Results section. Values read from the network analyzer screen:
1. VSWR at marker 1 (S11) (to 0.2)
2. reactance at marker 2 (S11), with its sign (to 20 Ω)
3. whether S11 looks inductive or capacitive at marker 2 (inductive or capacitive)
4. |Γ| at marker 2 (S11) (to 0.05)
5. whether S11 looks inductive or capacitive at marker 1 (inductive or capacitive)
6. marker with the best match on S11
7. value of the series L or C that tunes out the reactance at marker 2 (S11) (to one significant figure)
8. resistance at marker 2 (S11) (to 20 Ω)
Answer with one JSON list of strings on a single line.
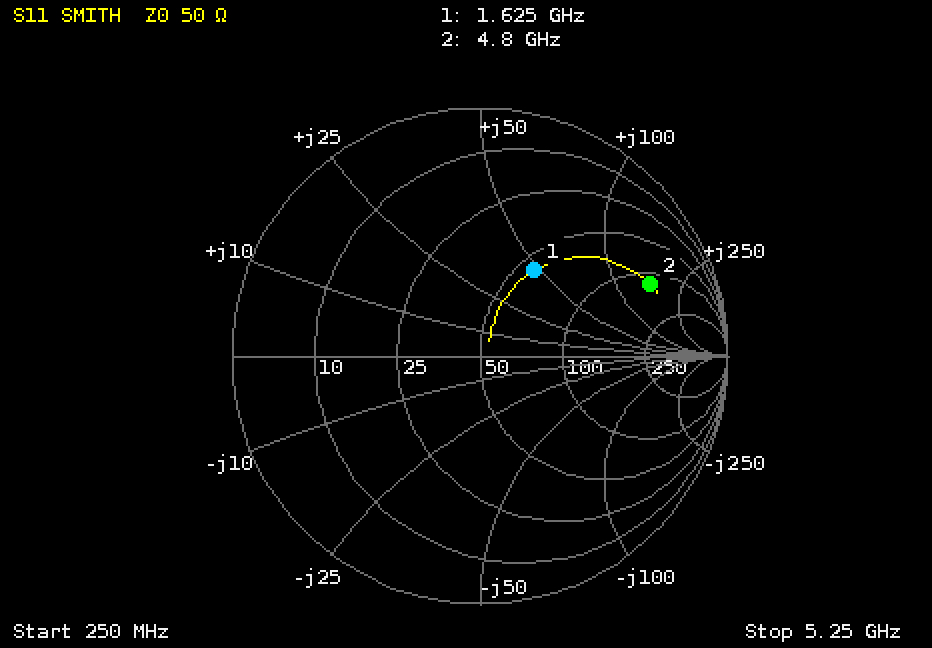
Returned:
["2.4", "+160 Ω", "inductive", "0.75", "inductive", "marker 1", "200 fF", "120 Ω"]
